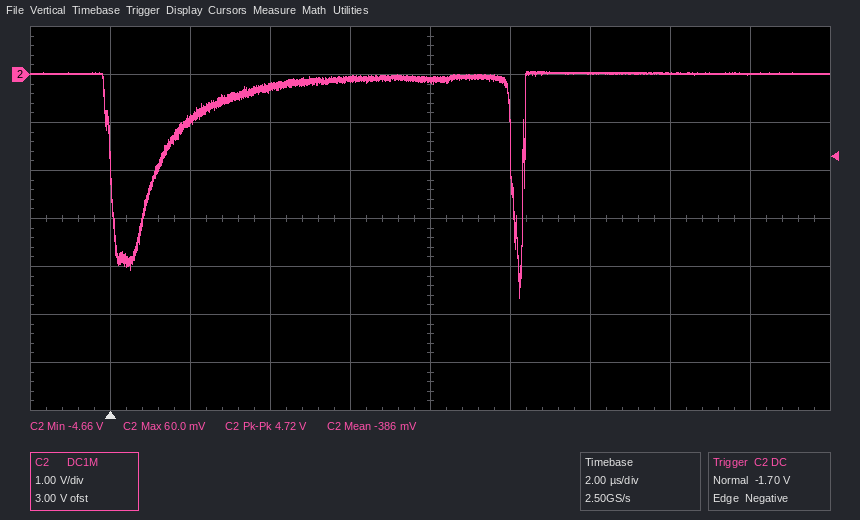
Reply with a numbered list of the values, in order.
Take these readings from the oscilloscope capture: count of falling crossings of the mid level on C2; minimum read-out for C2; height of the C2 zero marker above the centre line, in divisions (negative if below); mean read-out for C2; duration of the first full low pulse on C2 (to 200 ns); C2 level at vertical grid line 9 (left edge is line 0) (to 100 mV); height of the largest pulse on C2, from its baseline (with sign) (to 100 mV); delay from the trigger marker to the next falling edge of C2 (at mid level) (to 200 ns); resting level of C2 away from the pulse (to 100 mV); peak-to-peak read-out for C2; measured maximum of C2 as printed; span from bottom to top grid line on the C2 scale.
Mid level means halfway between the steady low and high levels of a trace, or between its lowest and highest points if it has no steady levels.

1. 2
2. -4.66 V
3. +3.0 div
4. -386 mV
5. 1.0 µs
6. 0.0 V
7. -4.7 V
8. 10.0 µs
9. 0.0 V
10. 4.72 V
11. 60.0 mV
12. 8 V
